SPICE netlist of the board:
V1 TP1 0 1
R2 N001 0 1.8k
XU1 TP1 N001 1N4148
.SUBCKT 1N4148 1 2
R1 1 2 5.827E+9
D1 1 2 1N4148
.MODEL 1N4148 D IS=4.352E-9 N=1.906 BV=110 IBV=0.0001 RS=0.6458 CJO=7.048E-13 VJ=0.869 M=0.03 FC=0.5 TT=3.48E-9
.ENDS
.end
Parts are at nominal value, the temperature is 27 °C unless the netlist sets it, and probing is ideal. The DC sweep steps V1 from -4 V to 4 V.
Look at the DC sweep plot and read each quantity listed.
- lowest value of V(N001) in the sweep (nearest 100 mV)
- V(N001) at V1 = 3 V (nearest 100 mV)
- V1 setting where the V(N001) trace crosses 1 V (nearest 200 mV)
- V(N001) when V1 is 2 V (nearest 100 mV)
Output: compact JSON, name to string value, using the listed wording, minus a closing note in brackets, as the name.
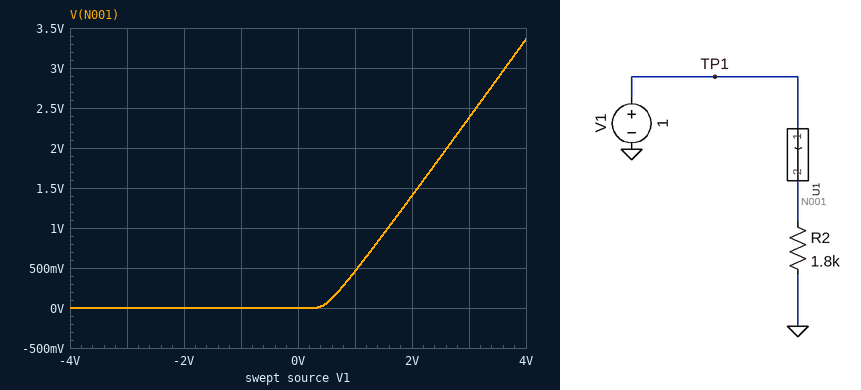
{"lowest value of V(N001) in the sweep": "0 V", "V(N001) at V1 = 3 V": "2.4 V", "V1 setting where the V(N001) trace crosses 1 V": "1.6 V", "V(N001) when V1 is 2 V": "1.4 V"}
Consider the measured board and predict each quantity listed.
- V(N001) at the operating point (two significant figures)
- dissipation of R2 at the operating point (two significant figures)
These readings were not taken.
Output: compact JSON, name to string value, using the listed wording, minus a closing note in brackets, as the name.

{"V(N001) at the operating point": "460 mV", "dissipation of R2 at the operating point": "120 µW"}
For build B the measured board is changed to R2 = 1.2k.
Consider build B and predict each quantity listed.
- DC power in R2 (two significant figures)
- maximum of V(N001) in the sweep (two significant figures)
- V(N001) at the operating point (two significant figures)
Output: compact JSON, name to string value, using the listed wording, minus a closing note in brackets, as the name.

{"DC power in R2": "160 µW", "maximum of V(N001) in the sweep": "3.3 V", "V(N001) at the operating point": "440 mV"}
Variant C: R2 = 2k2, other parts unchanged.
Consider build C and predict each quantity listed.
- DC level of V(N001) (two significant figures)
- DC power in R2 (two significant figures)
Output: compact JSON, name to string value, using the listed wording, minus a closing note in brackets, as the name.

{"DC level of V(N001)": "470 mV", "DC power in R2": "99 µW"}
